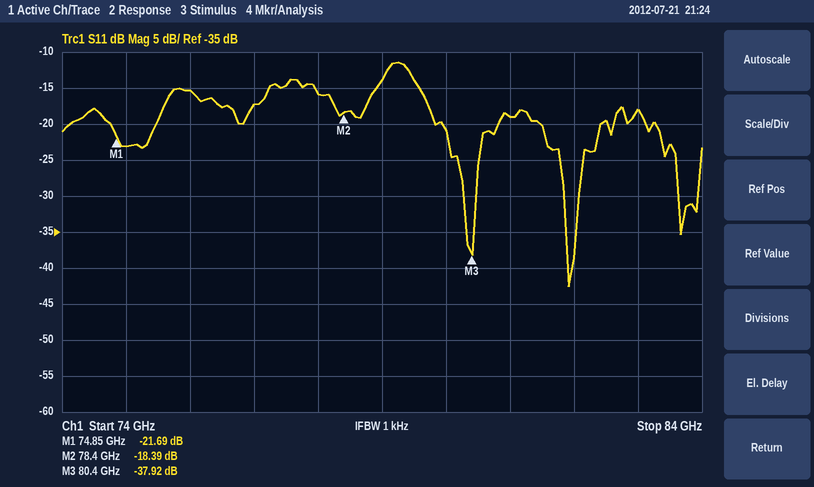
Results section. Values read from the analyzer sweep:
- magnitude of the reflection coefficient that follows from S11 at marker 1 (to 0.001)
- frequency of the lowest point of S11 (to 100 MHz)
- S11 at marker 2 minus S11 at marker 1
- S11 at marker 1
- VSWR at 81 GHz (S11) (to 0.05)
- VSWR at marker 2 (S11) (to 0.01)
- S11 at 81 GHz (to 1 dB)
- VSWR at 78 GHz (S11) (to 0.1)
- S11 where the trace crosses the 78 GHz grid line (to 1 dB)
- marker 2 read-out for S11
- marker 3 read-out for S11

0.082
81.9 GHz
3.30 dB
-21.69 dB
1.25
1.27
-19 dB
1.4
-16 dB
-18.39 dB
-37.92 dB
